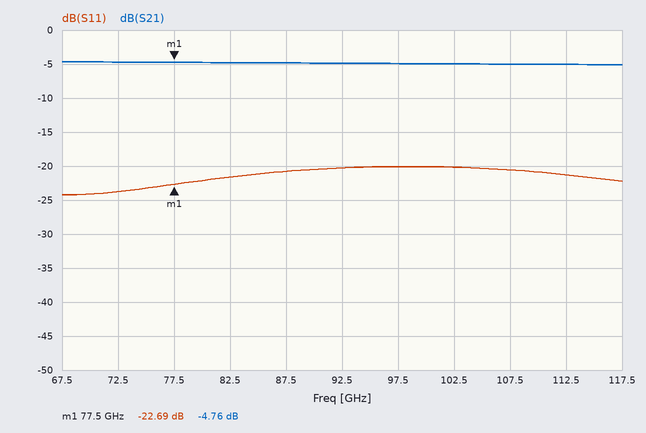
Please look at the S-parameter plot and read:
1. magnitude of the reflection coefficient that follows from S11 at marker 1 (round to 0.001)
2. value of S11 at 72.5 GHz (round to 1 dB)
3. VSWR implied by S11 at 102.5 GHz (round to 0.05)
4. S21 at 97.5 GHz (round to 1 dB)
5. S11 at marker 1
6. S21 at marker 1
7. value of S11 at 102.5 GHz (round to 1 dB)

0.073
-24 dB
1.20
-5 dB
-22.69 dB
-4.76 dB
-20 dB
